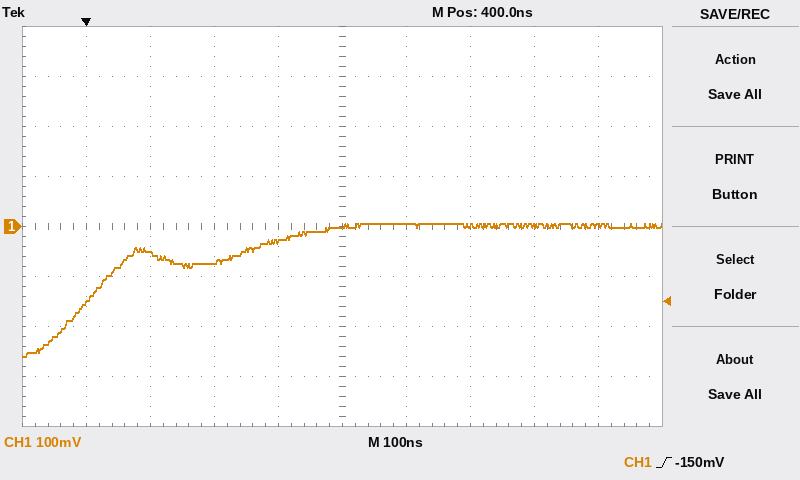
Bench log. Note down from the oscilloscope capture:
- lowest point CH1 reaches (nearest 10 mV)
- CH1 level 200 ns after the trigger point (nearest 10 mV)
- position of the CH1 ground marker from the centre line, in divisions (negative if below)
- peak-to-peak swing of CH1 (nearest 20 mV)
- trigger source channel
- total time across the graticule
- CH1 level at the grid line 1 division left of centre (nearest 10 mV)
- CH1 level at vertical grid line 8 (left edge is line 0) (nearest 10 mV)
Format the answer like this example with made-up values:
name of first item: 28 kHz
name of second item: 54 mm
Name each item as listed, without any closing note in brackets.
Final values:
lowest point CH1 reaches: -260 mV
CH1 level 200 ns after the trigger point: -70 mV
position of the CH1 ground marker from the centre line, in divisions: 0.0 div
peak-to-peak swing of CH1: 260 mV
trigger source channel: CH1
total time across the graticule: 1 µs
CH1 level at the grid line 1 division left of centre: -30 mV
CH1 level at vertical grid line 8 (left edge is line 0): 0 mV
